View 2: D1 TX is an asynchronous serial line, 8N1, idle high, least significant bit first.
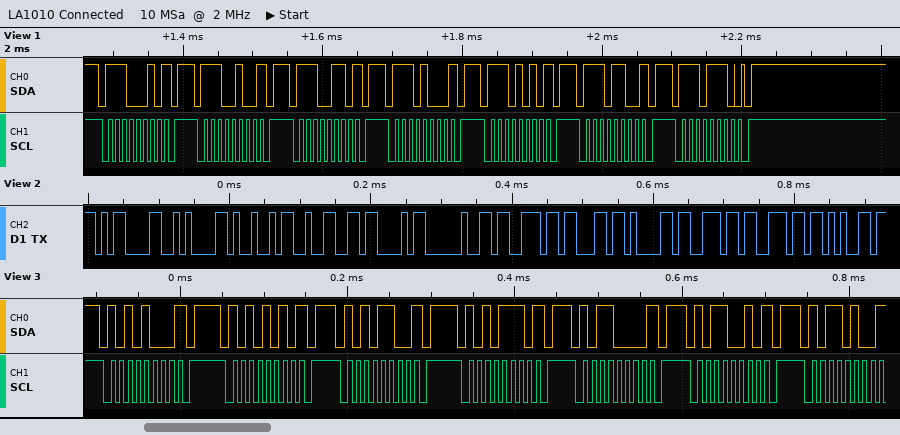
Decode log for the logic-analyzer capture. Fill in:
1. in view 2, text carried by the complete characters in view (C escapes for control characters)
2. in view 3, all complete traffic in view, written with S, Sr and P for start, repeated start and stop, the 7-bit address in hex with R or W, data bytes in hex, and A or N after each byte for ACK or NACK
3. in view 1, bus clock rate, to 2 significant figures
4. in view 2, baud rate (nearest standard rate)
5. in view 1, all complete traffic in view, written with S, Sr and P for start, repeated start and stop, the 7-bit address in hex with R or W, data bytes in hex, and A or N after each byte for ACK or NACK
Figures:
"\r\nI2C scanne"
S 54W N P S 55W N P S 56W N P S 57W N P S 58W N P S 59W N P S 5AW N
100 kHz
115200 baud
S 71W N P S 72W N P S 73W N P S 74W N P S 75W N P S 76W N P S 77W A P
